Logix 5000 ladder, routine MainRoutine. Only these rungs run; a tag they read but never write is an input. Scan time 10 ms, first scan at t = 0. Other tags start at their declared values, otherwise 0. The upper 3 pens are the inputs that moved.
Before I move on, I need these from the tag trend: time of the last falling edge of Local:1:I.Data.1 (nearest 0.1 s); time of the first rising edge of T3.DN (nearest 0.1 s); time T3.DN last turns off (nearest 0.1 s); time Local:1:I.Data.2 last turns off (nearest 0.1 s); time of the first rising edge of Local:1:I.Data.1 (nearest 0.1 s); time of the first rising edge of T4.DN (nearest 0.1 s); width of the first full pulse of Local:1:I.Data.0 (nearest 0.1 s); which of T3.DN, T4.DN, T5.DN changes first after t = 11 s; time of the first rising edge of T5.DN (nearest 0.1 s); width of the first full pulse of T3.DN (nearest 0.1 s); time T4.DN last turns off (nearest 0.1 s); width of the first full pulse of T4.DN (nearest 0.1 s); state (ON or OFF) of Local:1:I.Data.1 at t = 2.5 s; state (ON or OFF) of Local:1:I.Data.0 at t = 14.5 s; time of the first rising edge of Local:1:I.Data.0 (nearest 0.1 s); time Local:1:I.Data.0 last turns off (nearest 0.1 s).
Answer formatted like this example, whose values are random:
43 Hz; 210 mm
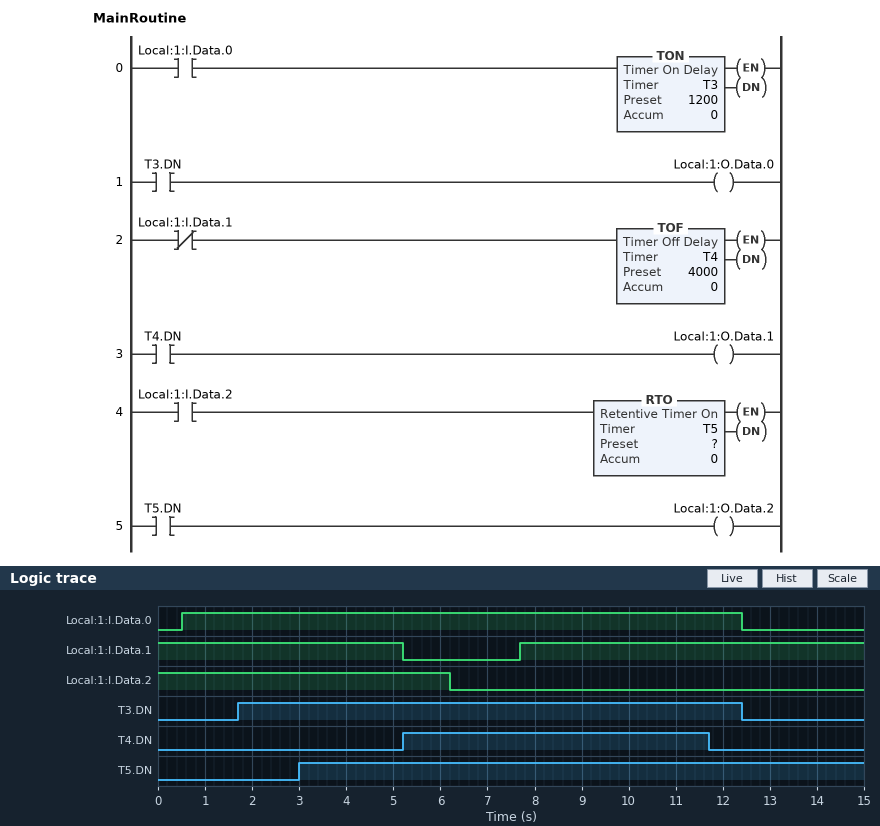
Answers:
5.2 s; 1.7 s; 12.4 s; 6.2 s; 7.7 s; 5.2 s; 11.9 s; T4.DN; 3.0 s; 10.7 s; 11.7 s; 6.5 s; ON; OFF; 0.5 s; 12.4 s
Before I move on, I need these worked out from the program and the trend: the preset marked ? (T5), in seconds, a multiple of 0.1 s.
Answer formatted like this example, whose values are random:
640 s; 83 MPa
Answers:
3.0 s
